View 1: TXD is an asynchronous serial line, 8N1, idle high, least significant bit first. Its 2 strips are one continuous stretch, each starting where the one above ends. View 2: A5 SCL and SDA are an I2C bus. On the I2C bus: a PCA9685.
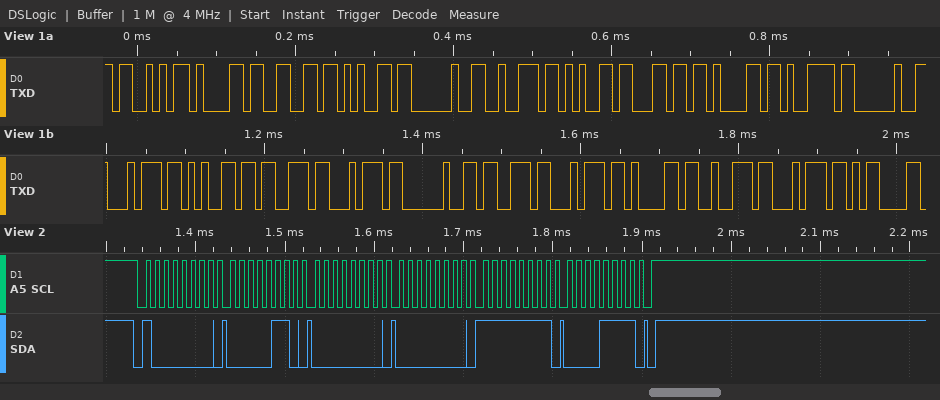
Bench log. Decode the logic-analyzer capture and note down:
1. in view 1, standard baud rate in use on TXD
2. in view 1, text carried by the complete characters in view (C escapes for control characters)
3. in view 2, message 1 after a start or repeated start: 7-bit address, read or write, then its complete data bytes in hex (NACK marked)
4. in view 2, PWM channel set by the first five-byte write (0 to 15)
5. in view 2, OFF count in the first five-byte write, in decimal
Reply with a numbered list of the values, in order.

1. 115200 baud
2. "Safe relay test start\r"
3. 0x40 write: 06 00 00 FF 0F
4. 0
5. 4095
